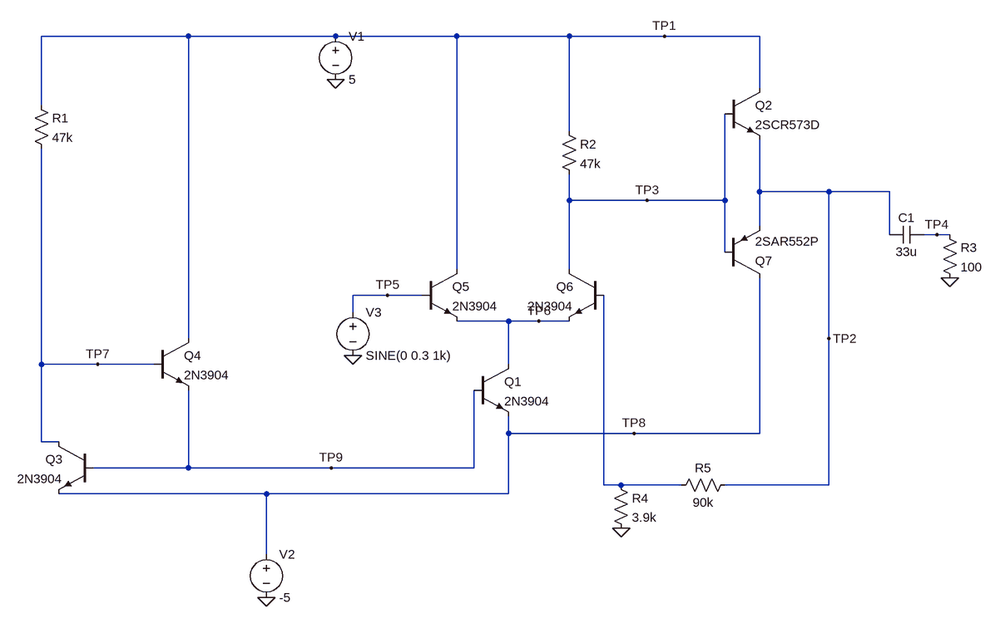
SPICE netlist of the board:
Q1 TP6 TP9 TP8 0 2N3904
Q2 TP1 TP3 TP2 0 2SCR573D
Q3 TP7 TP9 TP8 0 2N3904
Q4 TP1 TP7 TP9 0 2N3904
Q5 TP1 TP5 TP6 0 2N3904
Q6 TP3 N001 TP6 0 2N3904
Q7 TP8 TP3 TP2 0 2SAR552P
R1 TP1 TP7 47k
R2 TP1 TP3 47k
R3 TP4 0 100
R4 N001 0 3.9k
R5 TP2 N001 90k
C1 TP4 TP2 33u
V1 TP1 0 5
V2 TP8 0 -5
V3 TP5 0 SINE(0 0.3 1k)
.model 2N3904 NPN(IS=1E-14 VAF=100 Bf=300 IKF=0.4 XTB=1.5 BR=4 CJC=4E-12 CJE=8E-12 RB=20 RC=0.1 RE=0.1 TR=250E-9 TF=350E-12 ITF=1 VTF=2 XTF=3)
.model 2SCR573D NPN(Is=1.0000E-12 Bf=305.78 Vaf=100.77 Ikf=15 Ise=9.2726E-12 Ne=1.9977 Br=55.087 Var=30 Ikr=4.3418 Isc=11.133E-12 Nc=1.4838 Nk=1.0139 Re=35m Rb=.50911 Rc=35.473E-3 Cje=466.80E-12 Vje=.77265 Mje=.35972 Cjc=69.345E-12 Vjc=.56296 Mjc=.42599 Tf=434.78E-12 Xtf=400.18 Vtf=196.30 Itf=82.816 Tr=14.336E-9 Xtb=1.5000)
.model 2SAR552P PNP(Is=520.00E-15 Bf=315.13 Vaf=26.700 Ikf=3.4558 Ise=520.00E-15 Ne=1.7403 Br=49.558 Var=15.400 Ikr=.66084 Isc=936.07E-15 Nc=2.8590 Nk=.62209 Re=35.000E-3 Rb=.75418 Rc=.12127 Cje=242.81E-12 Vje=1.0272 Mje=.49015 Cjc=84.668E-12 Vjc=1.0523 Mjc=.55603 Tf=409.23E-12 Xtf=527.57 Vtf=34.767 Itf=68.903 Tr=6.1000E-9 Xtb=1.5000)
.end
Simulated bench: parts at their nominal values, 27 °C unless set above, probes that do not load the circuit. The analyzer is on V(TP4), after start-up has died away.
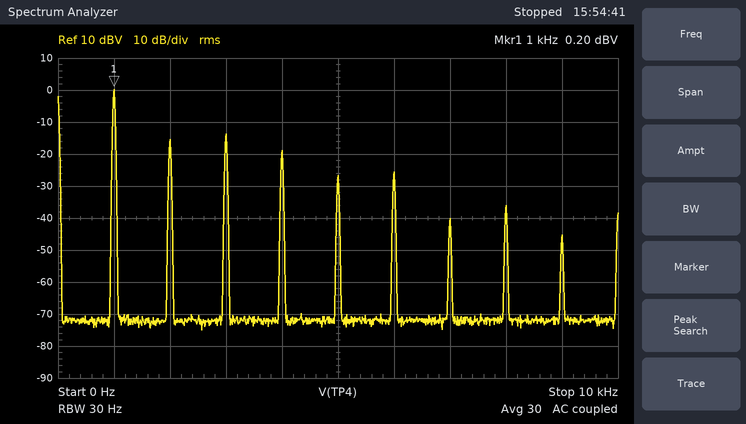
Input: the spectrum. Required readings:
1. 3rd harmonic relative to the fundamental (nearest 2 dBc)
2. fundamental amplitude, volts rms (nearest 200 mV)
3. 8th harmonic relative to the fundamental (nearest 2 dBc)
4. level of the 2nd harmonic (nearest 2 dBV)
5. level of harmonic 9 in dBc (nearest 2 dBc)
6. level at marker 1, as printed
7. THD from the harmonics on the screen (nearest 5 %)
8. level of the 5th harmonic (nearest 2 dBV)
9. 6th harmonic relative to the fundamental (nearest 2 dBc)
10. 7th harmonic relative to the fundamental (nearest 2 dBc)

-14 dBc
1.0 V
-36 dBc
-16 dBV
-46 dBc
0.20 dBV
30 %
-26 dBV
-26 dBc
-40 dBc
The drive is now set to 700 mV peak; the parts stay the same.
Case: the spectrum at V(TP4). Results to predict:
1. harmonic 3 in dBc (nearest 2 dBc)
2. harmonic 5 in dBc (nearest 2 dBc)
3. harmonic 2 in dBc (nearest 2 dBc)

-10 dBc
-16 dBc
-22 dBc
